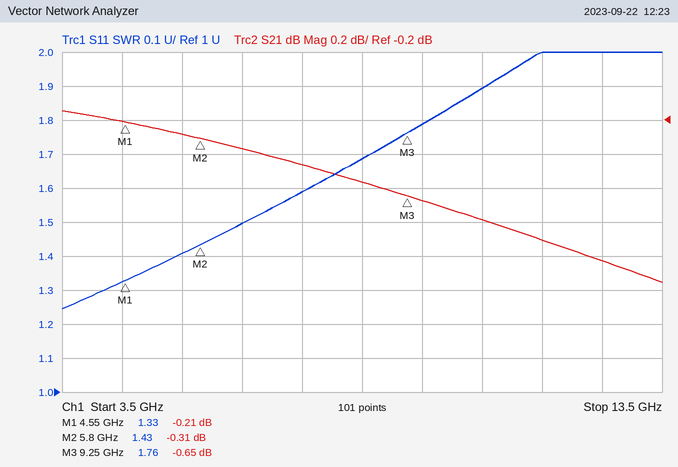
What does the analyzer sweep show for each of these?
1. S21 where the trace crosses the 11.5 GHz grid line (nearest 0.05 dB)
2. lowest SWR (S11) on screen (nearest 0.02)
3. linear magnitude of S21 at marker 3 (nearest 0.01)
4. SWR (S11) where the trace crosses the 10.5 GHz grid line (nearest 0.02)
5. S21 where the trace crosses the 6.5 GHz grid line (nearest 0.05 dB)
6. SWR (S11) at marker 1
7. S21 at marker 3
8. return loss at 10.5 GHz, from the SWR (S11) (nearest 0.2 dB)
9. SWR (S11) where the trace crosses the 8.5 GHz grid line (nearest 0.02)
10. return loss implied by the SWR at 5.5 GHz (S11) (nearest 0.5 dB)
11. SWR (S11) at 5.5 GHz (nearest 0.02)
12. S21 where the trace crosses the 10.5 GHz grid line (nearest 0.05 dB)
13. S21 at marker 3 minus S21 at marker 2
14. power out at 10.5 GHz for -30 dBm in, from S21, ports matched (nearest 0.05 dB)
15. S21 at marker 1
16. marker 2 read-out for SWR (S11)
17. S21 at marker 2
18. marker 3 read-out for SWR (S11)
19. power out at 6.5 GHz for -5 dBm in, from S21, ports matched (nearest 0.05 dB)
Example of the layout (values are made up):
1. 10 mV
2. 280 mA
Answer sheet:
1. -0.90 dB
2. 1.24
3. 0.93
4. 1.90
5. -0.35 dB
6. 1.33
7. -0.65 dB
8. 10.2 dB
9. 1.68
10. 15.5 dB
11. 1.40
12. -0.80 dB
13. -0.34 dB
14. -30.80 dBm
15. -0.21 dB
16. 1.43
17. -0.31 dB
18. 1.76
19. -5.35 dBm
